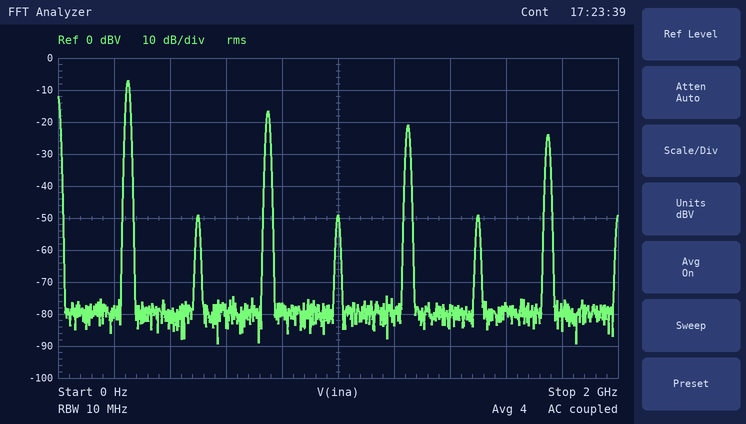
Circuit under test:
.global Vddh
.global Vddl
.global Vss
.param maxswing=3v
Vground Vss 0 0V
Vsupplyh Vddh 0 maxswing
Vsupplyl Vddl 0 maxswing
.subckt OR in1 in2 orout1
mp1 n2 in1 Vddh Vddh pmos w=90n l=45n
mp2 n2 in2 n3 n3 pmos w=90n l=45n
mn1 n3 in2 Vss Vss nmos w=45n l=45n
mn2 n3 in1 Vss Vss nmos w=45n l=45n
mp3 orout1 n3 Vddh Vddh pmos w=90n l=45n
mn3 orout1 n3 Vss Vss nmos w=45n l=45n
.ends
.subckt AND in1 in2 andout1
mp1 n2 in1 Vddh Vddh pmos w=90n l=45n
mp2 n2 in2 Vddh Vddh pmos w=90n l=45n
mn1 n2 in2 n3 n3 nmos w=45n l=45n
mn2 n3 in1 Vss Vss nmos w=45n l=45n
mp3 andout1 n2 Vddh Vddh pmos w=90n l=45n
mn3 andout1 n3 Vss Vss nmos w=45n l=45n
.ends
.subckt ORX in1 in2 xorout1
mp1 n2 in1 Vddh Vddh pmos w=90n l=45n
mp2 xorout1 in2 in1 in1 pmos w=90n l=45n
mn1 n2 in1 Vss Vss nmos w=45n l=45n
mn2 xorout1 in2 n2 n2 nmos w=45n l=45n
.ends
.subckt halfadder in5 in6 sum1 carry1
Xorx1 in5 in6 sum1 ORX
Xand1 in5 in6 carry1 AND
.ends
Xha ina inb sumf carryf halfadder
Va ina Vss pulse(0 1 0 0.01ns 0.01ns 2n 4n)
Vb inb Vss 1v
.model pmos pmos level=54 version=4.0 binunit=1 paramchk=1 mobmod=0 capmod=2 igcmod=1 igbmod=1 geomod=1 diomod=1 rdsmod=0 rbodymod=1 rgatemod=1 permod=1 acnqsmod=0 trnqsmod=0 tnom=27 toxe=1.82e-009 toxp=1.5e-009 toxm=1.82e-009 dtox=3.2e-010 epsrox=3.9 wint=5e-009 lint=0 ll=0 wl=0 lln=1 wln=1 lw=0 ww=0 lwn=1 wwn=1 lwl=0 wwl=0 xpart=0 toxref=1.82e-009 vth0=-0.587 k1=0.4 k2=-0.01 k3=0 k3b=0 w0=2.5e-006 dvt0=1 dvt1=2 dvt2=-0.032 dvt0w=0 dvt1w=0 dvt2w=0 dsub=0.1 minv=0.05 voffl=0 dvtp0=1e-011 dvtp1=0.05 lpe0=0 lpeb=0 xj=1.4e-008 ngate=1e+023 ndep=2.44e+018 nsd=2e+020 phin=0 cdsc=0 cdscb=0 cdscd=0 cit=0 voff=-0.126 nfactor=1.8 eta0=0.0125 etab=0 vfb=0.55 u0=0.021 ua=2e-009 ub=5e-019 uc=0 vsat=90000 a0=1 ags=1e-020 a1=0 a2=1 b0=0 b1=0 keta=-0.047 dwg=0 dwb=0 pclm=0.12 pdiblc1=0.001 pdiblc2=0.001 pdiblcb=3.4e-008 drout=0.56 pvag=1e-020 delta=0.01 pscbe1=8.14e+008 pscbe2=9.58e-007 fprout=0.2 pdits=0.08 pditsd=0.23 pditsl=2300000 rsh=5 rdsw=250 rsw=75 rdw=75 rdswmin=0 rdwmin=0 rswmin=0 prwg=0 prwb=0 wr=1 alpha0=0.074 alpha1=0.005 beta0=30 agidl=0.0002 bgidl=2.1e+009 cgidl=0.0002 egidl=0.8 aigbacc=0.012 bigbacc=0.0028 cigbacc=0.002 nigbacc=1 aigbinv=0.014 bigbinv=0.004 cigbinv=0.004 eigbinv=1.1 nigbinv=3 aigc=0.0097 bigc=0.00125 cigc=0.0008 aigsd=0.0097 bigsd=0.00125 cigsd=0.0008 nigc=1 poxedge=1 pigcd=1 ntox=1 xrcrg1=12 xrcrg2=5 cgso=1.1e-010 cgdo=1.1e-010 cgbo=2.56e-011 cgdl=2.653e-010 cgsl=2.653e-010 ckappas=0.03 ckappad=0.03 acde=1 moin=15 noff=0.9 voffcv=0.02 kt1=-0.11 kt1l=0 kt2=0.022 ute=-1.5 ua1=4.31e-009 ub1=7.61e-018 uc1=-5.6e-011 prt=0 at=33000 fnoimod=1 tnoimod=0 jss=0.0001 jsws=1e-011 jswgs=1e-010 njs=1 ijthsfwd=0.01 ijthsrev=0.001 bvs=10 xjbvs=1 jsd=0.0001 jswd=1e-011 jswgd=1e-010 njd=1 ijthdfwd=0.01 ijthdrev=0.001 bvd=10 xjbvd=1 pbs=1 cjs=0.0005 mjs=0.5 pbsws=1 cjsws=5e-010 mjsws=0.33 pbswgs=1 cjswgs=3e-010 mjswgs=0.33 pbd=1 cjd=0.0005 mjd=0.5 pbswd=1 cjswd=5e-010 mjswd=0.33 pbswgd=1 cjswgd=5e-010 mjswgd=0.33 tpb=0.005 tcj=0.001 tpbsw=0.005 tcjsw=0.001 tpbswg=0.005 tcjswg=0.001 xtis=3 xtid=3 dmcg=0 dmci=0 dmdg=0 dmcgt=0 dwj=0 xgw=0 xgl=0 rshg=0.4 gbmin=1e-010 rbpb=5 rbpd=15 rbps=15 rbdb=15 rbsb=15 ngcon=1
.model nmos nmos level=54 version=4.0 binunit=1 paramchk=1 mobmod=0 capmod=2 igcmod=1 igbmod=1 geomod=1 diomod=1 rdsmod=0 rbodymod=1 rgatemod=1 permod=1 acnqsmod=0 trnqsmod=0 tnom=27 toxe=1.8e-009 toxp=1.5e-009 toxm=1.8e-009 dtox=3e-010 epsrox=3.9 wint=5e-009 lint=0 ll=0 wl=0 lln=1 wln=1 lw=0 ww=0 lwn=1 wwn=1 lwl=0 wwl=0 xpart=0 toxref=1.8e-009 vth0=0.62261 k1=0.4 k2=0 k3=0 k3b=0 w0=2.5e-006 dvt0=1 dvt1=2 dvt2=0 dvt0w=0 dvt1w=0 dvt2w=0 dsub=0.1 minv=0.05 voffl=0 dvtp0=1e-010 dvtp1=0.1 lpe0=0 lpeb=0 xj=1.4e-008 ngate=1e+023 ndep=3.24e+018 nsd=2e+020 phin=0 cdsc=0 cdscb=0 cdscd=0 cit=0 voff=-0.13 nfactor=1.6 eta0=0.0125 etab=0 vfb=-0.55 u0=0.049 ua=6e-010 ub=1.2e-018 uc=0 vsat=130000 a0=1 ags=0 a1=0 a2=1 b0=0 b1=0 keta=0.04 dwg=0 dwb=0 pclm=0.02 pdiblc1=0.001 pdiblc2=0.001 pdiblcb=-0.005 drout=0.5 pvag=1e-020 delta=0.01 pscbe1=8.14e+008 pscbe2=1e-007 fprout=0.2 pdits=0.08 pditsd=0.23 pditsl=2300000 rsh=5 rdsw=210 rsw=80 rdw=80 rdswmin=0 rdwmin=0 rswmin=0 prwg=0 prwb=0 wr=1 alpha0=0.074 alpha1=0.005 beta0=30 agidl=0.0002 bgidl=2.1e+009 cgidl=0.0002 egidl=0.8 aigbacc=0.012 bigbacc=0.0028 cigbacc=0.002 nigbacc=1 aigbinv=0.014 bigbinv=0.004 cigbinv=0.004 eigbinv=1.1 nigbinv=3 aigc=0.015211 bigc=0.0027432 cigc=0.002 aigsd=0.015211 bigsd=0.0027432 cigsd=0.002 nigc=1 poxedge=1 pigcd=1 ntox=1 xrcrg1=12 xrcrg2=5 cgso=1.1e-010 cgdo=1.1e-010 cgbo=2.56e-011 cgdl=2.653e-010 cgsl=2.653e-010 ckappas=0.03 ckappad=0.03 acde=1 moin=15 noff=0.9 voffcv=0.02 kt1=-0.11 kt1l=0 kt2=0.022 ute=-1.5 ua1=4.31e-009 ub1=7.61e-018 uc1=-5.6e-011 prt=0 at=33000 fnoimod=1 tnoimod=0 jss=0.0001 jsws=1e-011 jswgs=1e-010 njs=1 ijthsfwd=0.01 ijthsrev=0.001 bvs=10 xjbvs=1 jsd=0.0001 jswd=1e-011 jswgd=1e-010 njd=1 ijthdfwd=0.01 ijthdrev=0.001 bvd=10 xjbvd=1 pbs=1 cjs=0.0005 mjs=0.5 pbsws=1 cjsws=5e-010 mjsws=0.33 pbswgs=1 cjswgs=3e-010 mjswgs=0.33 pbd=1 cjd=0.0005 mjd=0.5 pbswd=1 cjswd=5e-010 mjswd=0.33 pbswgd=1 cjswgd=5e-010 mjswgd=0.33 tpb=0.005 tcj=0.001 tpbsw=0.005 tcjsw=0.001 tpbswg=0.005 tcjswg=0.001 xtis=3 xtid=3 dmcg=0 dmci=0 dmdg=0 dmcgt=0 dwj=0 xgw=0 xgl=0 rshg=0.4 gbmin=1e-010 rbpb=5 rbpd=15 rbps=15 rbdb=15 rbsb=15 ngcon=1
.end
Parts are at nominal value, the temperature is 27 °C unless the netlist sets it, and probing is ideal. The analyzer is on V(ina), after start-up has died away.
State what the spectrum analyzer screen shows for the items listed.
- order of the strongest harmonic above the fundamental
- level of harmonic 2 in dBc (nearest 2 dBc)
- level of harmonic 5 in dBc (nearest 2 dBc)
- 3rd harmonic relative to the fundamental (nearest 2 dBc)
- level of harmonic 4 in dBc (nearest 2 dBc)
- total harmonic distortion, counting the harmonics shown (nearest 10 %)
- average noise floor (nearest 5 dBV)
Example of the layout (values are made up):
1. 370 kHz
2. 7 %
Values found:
1. 3
2. -42 dBc
3. -14 dBc
4. -10 dBc
5. -42 dBc
6. 40 %
7. -80 dBV
